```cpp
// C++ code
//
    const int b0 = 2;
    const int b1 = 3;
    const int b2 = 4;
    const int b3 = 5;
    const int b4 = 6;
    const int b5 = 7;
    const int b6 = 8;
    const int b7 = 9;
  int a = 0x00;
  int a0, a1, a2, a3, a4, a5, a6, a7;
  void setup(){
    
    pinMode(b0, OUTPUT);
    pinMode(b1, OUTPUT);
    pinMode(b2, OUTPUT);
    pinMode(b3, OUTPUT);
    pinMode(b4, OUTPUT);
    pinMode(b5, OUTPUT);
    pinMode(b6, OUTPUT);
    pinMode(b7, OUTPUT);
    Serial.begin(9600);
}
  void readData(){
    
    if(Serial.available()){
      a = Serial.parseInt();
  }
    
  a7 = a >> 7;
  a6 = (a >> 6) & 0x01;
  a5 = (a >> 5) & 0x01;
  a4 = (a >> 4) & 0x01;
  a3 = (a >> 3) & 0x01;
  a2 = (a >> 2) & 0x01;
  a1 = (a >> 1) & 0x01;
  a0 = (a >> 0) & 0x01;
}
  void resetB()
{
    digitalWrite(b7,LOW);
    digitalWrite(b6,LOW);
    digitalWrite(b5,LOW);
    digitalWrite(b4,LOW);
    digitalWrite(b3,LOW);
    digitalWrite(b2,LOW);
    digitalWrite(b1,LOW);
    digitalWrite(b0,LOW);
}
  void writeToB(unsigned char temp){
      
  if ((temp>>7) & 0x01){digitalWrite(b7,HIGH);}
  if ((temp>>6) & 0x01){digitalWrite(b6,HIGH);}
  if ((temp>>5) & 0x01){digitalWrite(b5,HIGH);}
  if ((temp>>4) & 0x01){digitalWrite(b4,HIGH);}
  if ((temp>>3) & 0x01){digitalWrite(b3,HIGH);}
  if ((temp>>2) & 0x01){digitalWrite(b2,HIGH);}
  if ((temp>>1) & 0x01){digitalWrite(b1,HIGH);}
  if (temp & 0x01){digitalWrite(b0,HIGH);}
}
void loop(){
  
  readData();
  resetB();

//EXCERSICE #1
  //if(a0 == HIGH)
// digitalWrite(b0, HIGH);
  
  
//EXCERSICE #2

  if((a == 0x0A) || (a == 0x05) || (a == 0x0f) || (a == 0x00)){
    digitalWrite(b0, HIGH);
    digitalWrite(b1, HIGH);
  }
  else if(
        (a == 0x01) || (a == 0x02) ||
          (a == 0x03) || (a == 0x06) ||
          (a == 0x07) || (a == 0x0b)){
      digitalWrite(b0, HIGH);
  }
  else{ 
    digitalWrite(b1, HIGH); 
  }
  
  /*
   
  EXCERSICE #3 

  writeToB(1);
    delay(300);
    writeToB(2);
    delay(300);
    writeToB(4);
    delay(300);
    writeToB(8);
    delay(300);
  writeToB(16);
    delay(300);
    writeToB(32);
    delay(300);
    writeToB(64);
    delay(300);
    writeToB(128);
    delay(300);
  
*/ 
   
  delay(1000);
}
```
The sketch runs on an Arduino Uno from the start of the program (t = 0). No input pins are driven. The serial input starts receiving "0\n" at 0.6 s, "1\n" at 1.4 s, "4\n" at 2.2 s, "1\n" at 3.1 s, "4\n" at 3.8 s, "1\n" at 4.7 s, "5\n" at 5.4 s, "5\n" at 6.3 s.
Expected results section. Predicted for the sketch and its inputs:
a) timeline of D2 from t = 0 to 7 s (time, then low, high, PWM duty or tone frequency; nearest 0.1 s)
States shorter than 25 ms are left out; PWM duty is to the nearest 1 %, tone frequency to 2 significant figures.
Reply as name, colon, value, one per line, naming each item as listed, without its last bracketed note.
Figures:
timeline of D2 from t = 0 to 7 s: 0 s high; 3 s low; 4 s high; 5 s low; 6 s high
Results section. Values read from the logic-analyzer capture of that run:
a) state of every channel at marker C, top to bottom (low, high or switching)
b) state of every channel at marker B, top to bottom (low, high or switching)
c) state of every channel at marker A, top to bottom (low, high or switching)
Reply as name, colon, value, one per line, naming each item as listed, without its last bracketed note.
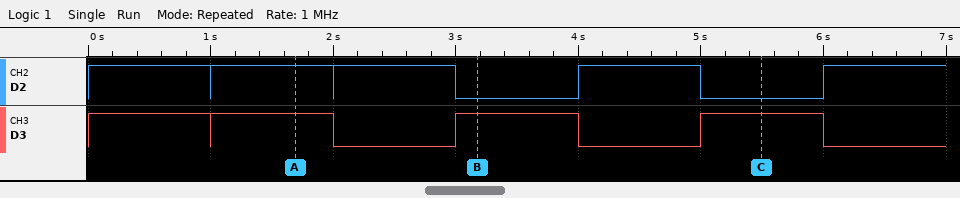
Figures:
state of every channel at marker C, top to bottom: D2 low, D3 high
state of every channel at marker B, top to bottom: D2 low, D3 high
state of every channel at marker A, top to bottom: D2 high, D3 high
